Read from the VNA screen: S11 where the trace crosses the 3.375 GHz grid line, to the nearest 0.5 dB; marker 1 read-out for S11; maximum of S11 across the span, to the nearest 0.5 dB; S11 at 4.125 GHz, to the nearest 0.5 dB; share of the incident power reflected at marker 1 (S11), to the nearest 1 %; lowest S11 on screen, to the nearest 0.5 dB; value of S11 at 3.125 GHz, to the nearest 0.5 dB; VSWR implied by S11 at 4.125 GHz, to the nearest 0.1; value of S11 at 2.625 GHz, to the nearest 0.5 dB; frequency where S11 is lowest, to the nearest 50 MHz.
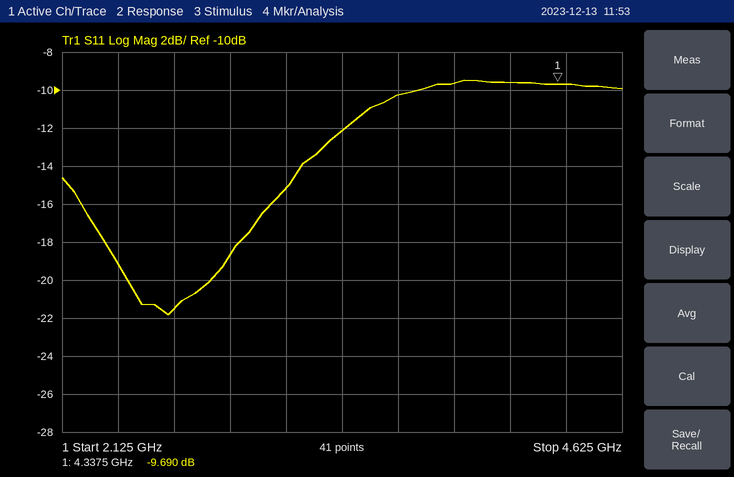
-12.0 dB
-9.690 dB
-9.5 dB
-9.5 dB
11 %
-22.0 dB
-15.0 dB
2.0
-21.5 dB
2.60 GHz
